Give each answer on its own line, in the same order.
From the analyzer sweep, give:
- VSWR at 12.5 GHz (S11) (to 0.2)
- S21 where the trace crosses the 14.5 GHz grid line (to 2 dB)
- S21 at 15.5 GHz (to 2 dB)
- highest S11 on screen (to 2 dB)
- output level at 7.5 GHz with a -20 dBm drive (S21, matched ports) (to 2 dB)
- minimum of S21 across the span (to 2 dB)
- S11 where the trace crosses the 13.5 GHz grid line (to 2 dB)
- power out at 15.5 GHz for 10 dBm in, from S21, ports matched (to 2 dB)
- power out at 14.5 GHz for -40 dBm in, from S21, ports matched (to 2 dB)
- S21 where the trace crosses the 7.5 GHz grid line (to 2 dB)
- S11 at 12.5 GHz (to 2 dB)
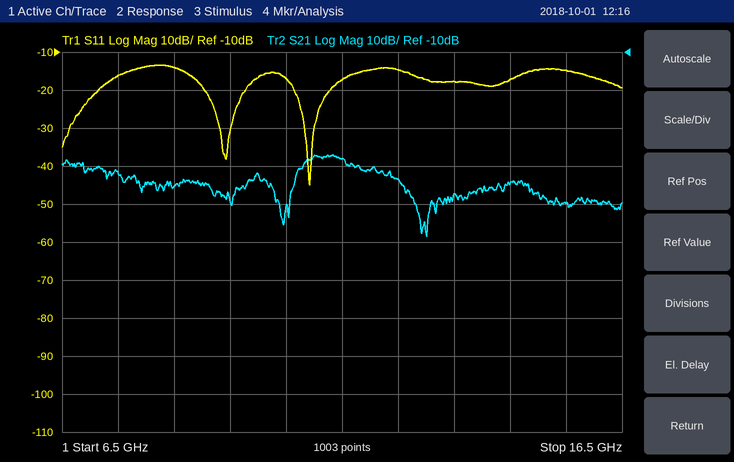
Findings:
1.4
-44 dB
-50 dB
-14 dB
-62 dBm
-58 dB
-18 dB
-40 dBm
-84 dBm
-42 dB
-14 dB
